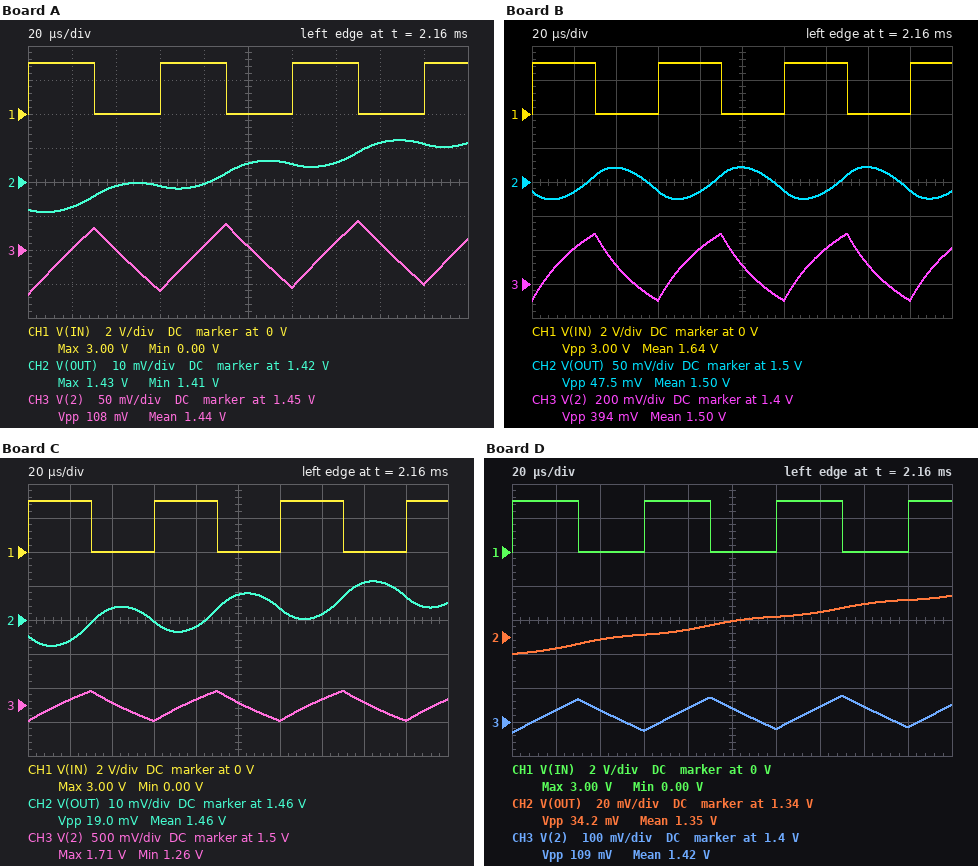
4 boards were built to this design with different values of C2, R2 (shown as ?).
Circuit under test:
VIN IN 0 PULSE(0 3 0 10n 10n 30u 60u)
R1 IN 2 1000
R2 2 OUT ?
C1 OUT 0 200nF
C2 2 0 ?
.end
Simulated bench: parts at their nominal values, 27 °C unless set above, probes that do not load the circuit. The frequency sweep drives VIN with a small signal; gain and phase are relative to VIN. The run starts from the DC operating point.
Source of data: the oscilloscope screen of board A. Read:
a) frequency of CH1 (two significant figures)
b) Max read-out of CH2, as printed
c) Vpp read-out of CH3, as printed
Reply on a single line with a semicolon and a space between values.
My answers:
17 kHz; 1.43 V; 108 mV
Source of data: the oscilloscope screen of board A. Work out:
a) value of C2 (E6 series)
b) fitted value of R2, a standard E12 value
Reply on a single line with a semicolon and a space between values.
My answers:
470 nF; 820 Ω
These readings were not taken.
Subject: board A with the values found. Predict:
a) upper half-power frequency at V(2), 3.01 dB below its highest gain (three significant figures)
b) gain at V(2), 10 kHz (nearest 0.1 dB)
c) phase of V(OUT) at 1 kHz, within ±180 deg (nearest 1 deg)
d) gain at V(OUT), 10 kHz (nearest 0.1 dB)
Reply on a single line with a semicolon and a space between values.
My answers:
225 Hz; -29.5 dB; -111 deg; -49.8 dB
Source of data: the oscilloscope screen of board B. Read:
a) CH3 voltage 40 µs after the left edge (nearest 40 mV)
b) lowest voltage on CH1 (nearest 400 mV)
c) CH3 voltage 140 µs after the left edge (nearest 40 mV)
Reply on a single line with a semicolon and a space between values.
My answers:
1.52 V; 0 V; 1.60 V
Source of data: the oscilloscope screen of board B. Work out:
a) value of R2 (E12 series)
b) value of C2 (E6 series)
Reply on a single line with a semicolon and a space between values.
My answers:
330 Ω; 100 nF
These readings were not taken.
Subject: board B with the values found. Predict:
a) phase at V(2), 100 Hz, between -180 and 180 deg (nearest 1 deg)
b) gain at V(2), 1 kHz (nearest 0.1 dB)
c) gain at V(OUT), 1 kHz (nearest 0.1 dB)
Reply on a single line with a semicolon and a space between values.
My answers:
-11 deg; -7.0 dB; -7.7 dB
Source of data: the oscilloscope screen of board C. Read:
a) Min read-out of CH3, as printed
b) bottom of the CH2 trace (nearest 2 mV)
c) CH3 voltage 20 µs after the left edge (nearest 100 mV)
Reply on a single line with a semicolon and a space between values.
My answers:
1.26 V; 1.452 V; 1.6 V
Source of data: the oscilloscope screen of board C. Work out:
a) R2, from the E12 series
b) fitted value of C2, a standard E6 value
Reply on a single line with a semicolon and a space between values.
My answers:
1.8 kΩ; 100 nF
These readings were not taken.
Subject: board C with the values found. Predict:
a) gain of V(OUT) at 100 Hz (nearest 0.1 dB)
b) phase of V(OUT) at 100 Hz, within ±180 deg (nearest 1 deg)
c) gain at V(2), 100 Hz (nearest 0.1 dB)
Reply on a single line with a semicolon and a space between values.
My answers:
-0.6 dB; -23 deg; -0.4 dB
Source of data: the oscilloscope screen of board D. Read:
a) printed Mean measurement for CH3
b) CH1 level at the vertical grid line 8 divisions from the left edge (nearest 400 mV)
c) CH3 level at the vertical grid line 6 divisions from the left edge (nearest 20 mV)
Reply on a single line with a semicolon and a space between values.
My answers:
1.42 V; 0 V; 1.38 V
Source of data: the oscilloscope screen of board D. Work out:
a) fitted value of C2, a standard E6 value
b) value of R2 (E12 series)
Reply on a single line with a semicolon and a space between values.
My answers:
470 nF; 2.2 kΩ
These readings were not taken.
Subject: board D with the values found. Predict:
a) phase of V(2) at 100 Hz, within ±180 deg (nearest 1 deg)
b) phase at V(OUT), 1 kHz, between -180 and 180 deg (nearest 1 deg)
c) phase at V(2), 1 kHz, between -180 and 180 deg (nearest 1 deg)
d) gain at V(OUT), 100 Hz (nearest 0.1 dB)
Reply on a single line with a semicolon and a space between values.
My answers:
-22 deg; -136 deg; -66 deg; -1.2 dB
